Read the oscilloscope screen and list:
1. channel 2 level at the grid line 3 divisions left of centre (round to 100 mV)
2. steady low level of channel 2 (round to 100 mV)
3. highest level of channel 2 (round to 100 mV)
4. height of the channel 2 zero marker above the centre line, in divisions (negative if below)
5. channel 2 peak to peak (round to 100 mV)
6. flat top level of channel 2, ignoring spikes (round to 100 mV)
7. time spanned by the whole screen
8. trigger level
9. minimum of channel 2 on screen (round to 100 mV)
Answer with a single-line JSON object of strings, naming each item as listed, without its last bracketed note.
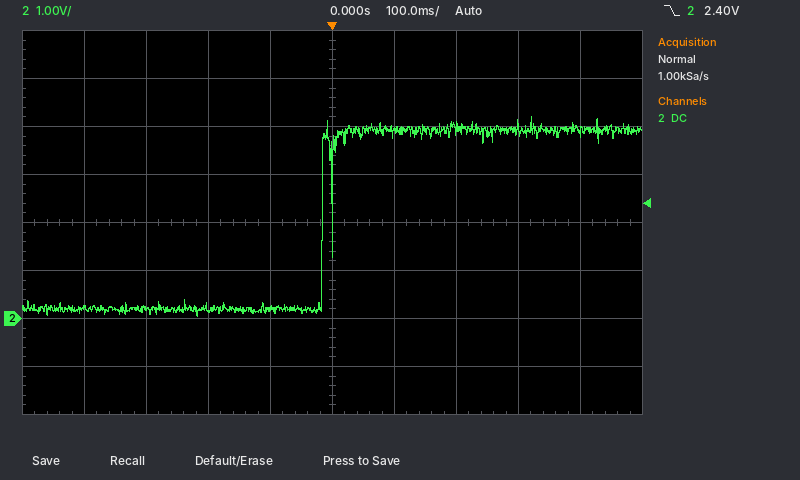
{"channel 2 level at the grid line 3 divisions left of centre": "200 mV", "steady low level of channel 2": "200 mV", "highest level of channel 2": "4.2 V", "height of the channel 2 zero marker above the centre line, in divisions": "-2.0 div", "channel 2 peak to peak": "4.2 V", "flat top level of channel 2, ignoring spikes": "3.9 V", "time spanned by the whole screen": "1 s", "trigger level": "2.40 V", "minimum of channel 2 on screen": "0.0 V"}
